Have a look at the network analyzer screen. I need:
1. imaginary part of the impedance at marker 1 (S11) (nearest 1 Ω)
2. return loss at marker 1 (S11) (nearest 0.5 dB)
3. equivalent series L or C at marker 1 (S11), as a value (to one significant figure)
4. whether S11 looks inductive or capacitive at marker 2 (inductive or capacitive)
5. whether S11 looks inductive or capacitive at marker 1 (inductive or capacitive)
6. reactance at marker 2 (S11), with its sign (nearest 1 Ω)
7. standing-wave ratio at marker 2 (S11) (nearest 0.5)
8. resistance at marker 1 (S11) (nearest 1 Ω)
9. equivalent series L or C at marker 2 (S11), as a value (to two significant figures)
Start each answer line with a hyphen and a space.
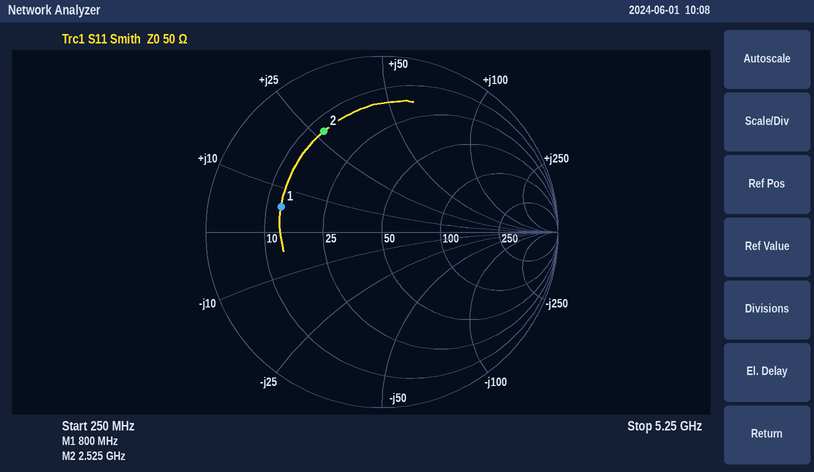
- +6 Ω
- 4.5 dB
- 1 nH
- inductive
- inductive
- +27 Ω
- 5.0
- 13 Ω
- 1.7 nH
